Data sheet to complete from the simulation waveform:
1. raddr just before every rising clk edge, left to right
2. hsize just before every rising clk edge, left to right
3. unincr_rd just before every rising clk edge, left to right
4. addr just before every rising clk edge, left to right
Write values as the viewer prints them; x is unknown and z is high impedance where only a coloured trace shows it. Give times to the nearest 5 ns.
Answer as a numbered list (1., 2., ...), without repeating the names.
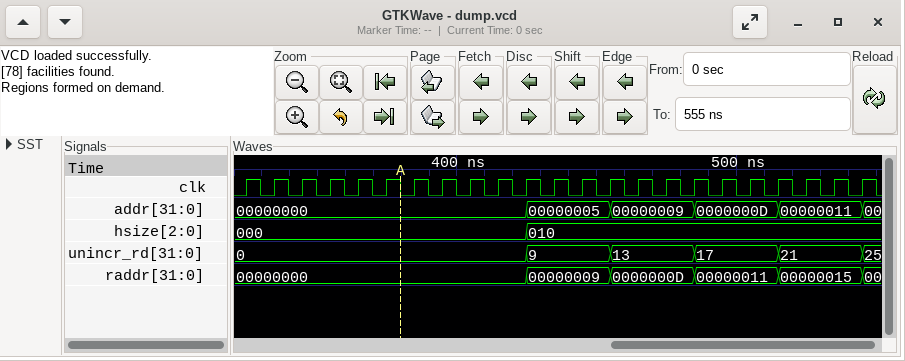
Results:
1. 00000000, 00000000, 00000000, 00000000, 00000000, 00000000, 00000000, 00000000, 00000000, 00000000, 00000000, 00000009, 00000009, 00000009, 0000000D, 0000000D, 0000000D, 00000011, 00000011, 00000011, 00000015, 00000015, 00000015
2. 000, 000, 000, 000, 000, 000, 000, 000, 000, 000, 000, 010, 010, 010, 010, 010, 010, 010, 010, 010, 010, 010, 010
3. 0, 0, 0, 0, 0, 0, 0, 0, 0, 0, 0, 9, 9, 9, 13, 13, 13, 17, 17, 17, 21, 21, 21
4. 00000000, 00000000, 00000000, 00000000, 00000000, 00000000, 00000000, 00000000, 00000000, 00000000, 00000000, 00000005, 00000005, 00000005, 00000009, 00000009, 00000009, 0000000D, 0000000D, 0000000D, 00000011, 00000011, 00000011
